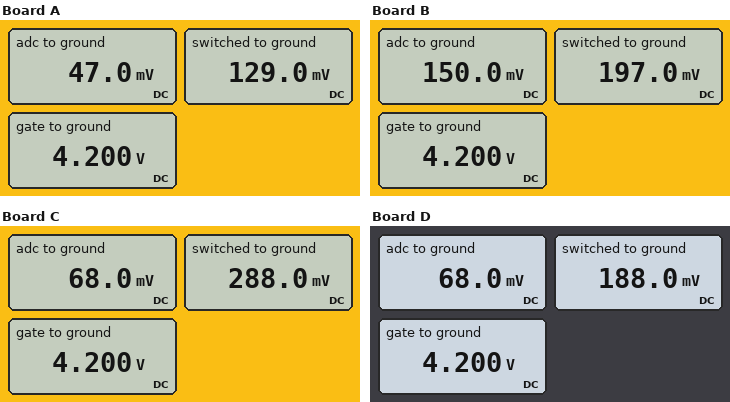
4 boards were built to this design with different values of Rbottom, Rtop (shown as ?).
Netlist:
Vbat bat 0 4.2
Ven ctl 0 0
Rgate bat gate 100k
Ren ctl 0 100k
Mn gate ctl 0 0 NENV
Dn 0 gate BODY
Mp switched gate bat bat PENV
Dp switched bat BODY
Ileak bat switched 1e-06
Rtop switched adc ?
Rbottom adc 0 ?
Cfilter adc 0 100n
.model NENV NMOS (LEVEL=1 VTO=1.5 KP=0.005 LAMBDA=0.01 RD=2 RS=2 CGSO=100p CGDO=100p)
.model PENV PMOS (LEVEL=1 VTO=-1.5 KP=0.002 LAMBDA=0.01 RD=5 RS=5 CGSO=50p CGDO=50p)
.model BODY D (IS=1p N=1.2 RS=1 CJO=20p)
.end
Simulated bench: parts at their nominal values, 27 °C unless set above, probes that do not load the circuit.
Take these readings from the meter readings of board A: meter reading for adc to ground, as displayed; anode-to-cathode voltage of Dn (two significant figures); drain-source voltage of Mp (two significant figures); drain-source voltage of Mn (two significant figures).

47.0 mV
-4.2 V
-4.1 V
4.2 V
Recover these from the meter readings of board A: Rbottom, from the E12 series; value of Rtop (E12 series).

47 kΩ
82 kΩ
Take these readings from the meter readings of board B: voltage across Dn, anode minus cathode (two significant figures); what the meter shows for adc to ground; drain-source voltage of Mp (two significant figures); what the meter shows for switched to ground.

-4.2 V
150.0 mV
-4.0 V
197.0 mV
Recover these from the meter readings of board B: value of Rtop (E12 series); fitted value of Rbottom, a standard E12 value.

47 kΩ
150 kΩ
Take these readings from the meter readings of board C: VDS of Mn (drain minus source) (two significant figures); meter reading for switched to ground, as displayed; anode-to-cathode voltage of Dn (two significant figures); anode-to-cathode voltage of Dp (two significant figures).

4.2 V
288.0 mV
-4.2 V
-3.9 V
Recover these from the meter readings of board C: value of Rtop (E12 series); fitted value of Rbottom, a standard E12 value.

220 kΩ
68 kΩ
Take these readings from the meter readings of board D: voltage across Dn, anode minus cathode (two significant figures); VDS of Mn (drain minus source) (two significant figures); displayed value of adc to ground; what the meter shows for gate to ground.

-4.2 V
4.2 V
68.0 mV
4.200 V
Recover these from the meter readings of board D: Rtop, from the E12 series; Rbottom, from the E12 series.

120 kΩ
68 kΩ
